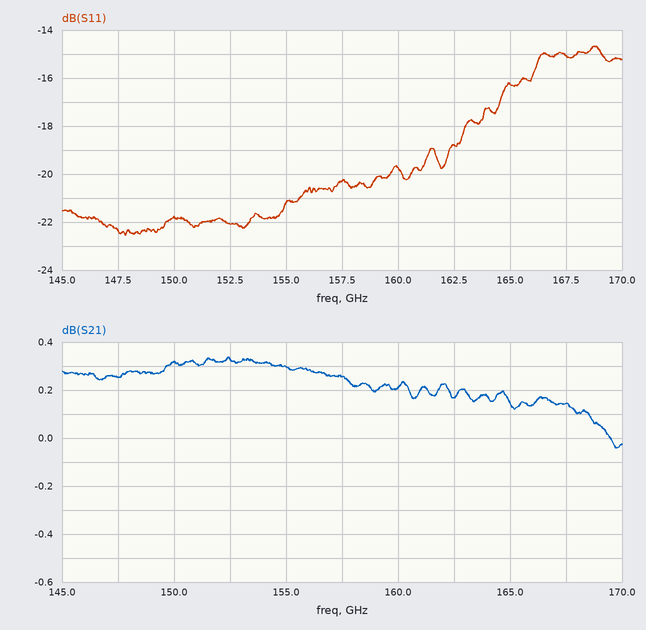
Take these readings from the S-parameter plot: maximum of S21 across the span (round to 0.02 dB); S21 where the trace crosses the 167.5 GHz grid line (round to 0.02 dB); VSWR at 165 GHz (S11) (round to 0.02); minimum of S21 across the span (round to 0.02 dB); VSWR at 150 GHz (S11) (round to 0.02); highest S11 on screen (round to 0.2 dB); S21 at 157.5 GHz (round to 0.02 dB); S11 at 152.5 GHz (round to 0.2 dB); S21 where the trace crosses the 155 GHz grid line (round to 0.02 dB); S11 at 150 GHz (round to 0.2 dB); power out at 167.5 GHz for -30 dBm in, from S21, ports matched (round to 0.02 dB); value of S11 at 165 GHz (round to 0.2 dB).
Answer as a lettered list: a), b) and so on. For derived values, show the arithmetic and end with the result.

a) 0.34 dB
b) 0.14 dB
c) |Γ| = 10^(-16.2/20) = 0.1549; VSWR = (1 + 0.1549)/(1 − 0.1549) ≈ 1.37, so 1.36 to the nearest 0.02
d) -0.04 dB
e) |Γ| = 10^(-21.8/20) = 0.0813; VSWR = (1 + 0.0813)/(1 − 0.0813) ≈ 1.18
f) -14.6 dB
g) 0.26 dB
h) -22.0 dB
i) 0.30 dB
j) -21.8 dB
k) -30 dBm + (0.14 dB) = -29.86 dBm
l) -16.2 dB
